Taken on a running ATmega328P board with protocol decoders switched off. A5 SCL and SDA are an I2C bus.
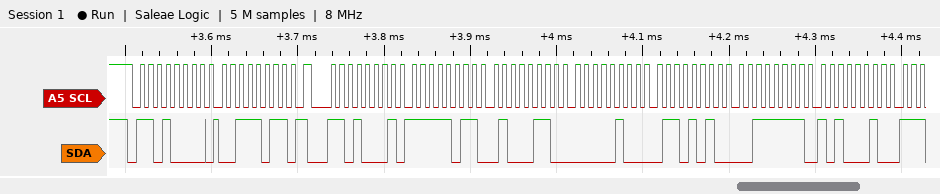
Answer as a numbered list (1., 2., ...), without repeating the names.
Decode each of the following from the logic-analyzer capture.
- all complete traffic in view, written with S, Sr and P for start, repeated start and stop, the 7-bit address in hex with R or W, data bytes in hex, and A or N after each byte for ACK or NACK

1. S 68W A 3B A Sr 68R A FB A 46 A 04 A 6A A 3F A A2 A
